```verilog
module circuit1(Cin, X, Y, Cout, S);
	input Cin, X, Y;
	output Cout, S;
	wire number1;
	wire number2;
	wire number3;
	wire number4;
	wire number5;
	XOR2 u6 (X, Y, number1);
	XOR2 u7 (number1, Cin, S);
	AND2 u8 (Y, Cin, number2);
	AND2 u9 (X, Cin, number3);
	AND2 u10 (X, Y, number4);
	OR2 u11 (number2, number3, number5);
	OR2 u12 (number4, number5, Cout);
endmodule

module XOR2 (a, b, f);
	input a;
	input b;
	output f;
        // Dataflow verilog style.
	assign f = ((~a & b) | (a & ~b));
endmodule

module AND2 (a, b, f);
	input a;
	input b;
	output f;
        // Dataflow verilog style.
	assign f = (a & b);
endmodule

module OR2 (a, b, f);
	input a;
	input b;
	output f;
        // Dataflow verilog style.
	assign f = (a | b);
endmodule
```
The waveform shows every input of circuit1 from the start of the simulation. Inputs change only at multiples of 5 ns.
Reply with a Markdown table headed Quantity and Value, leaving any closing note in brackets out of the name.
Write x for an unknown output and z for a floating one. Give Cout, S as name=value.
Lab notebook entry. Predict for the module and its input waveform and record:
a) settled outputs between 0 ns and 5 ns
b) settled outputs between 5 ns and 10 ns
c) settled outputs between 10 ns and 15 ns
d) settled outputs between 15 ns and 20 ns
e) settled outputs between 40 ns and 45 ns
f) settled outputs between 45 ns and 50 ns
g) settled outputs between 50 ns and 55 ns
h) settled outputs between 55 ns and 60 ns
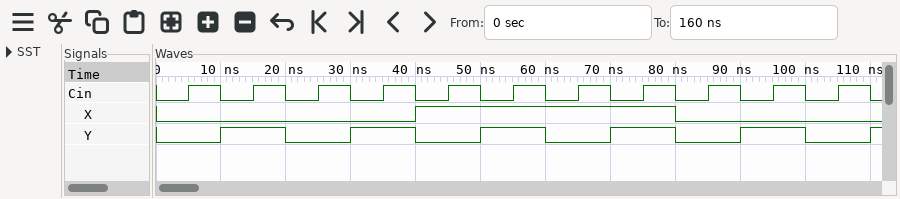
| Quantity | Value |
|---|---|
| settled outputs between 0 ns and 5 ns | Cout=0, S=0 |
| settled outputs between 5 ns and 10 ns | Cout=0, S=1 |
| settled outputs between 10 ns and 15 ns | Cout=0, S=1 |
| settled outputs between 15 ns and 20 ns | Cout=1, S=0 |
| settled outputs between 40 ns and 45 ns | Cout=0, S=1 |
| settled outputs between 45 ns and 50 ns | Cout=1, S=0 |
| settled outputs between 50 ns and 55 ns | Cout=1, S=0 |
| settled outputs between 55 ns and 60 ns | Cout=1, S=1 |
